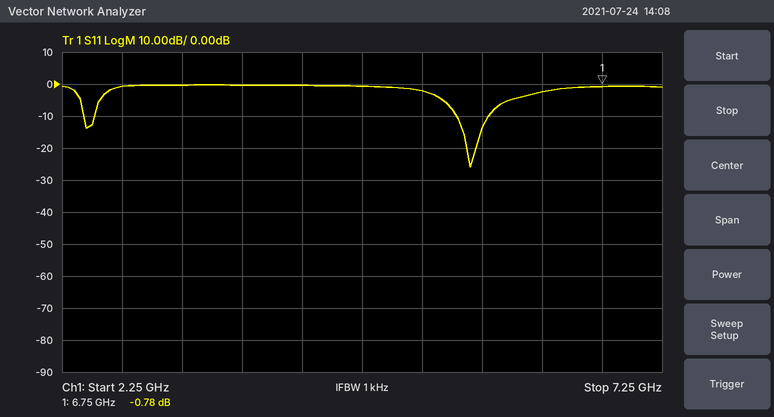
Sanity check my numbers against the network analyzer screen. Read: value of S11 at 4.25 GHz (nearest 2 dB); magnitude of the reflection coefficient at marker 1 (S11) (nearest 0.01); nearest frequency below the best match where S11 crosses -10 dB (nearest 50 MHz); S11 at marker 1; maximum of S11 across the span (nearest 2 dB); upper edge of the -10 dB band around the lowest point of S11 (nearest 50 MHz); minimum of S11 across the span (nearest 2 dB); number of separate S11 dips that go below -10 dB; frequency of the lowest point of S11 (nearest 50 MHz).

0 dB
0.91
5.55 GHz
-0.78 dB
0 dB
5.80 GHz
-26 dB
2
5.65 GHz
